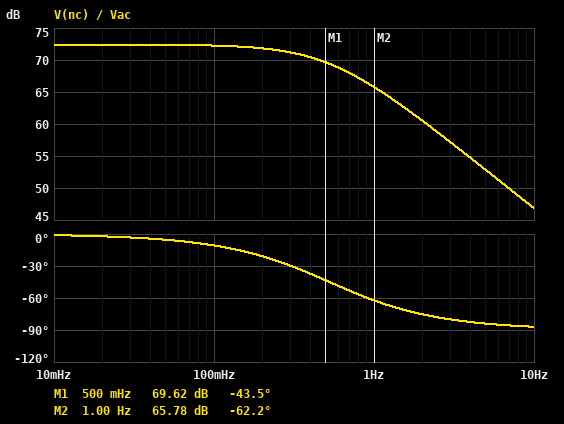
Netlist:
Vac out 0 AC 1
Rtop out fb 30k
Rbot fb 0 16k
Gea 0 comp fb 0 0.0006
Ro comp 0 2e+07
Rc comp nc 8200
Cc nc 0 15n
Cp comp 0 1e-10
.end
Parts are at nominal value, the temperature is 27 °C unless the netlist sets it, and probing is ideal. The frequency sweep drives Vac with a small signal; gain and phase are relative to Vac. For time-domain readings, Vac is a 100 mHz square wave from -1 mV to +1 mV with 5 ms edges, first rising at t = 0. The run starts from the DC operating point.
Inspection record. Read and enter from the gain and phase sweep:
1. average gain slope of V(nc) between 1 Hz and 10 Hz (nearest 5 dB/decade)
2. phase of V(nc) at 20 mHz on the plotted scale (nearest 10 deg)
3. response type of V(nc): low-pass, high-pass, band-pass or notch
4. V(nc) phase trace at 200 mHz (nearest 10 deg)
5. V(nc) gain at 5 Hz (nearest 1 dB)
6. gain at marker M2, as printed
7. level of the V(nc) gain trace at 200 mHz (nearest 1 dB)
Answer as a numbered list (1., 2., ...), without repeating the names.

1. -20 dB/decade
2. 0 deg
3. low-pass
4. -20 deg
5. 53 dB
6. 65.78 dB
7. 72 dB
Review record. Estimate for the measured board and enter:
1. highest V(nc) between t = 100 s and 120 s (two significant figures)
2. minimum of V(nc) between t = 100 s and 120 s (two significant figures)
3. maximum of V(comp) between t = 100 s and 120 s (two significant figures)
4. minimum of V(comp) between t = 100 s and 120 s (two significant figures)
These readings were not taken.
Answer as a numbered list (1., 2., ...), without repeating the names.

1. 4.2 V
2. -4.2 V
3. 4.2 V
4. -4.2 V
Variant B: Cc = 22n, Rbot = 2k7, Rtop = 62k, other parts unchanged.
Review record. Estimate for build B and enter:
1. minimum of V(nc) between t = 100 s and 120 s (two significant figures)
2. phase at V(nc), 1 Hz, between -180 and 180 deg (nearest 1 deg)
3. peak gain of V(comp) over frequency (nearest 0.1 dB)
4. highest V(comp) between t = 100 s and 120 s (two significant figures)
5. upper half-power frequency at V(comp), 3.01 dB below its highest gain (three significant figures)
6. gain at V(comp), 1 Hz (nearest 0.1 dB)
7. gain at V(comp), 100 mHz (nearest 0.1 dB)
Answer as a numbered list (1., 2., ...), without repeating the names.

1. -500 mV
2. -70 deg
3. 54.0 dB
4. 500 mV
5. 360 mHz
6. 44.6 dB
7. 53.7 dB
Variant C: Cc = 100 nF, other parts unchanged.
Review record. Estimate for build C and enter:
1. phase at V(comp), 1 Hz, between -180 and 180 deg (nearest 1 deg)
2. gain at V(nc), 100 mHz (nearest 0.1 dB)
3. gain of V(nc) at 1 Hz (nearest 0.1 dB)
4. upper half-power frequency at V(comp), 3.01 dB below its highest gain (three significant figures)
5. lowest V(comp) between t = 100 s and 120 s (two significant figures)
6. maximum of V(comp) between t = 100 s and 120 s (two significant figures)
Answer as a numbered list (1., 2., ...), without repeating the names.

1. -85 deg
2. 68.3 dB
3. 50.4 dB
4. 79.5 mHz
5. -3.5 V
6. 3.5 V
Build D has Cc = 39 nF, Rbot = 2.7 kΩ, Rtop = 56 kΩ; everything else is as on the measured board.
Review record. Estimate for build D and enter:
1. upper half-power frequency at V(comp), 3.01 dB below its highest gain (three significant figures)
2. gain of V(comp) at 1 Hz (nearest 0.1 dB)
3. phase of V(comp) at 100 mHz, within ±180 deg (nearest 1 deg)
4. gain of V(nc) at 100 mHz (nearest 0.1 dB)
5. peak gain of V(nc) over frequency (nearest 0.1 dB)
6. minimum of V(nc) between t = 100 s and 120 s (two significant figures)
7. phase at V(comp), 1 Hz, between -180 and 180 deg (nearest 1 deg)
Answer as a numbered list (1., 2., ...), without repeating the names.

1. 203 mHz
2. 40.8 dB
3. -26 deg
4. 53.9 dB
5. 54.8 dB
6. -550 mV
7. -78 deg
